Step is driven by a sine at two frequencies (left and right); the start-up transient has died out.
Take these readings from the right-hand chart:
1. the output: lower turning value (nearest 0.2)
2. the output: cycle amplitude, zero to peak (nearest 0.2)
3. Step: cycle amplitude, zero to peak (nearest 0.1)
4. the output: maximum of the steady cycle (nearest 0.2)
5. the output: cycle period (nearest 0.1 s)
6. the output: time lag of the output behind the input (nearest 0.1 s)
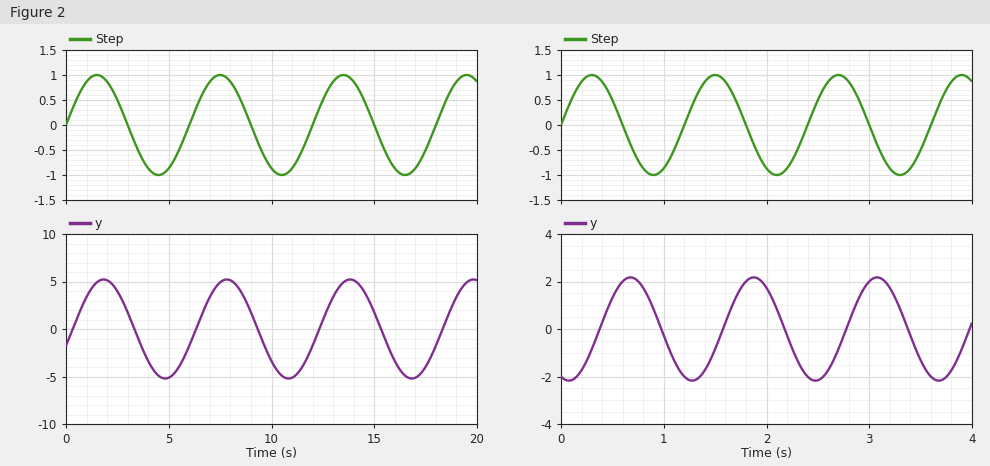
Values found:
-2.2
2.2
1.0
2.2
1.2 s
0.4 s
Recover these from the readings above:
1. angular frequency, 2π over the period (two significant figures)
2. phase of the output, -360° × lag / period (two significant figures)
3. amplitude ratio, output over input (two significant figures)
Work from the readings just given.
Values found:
5.2 rad/s
-120°
2.2
